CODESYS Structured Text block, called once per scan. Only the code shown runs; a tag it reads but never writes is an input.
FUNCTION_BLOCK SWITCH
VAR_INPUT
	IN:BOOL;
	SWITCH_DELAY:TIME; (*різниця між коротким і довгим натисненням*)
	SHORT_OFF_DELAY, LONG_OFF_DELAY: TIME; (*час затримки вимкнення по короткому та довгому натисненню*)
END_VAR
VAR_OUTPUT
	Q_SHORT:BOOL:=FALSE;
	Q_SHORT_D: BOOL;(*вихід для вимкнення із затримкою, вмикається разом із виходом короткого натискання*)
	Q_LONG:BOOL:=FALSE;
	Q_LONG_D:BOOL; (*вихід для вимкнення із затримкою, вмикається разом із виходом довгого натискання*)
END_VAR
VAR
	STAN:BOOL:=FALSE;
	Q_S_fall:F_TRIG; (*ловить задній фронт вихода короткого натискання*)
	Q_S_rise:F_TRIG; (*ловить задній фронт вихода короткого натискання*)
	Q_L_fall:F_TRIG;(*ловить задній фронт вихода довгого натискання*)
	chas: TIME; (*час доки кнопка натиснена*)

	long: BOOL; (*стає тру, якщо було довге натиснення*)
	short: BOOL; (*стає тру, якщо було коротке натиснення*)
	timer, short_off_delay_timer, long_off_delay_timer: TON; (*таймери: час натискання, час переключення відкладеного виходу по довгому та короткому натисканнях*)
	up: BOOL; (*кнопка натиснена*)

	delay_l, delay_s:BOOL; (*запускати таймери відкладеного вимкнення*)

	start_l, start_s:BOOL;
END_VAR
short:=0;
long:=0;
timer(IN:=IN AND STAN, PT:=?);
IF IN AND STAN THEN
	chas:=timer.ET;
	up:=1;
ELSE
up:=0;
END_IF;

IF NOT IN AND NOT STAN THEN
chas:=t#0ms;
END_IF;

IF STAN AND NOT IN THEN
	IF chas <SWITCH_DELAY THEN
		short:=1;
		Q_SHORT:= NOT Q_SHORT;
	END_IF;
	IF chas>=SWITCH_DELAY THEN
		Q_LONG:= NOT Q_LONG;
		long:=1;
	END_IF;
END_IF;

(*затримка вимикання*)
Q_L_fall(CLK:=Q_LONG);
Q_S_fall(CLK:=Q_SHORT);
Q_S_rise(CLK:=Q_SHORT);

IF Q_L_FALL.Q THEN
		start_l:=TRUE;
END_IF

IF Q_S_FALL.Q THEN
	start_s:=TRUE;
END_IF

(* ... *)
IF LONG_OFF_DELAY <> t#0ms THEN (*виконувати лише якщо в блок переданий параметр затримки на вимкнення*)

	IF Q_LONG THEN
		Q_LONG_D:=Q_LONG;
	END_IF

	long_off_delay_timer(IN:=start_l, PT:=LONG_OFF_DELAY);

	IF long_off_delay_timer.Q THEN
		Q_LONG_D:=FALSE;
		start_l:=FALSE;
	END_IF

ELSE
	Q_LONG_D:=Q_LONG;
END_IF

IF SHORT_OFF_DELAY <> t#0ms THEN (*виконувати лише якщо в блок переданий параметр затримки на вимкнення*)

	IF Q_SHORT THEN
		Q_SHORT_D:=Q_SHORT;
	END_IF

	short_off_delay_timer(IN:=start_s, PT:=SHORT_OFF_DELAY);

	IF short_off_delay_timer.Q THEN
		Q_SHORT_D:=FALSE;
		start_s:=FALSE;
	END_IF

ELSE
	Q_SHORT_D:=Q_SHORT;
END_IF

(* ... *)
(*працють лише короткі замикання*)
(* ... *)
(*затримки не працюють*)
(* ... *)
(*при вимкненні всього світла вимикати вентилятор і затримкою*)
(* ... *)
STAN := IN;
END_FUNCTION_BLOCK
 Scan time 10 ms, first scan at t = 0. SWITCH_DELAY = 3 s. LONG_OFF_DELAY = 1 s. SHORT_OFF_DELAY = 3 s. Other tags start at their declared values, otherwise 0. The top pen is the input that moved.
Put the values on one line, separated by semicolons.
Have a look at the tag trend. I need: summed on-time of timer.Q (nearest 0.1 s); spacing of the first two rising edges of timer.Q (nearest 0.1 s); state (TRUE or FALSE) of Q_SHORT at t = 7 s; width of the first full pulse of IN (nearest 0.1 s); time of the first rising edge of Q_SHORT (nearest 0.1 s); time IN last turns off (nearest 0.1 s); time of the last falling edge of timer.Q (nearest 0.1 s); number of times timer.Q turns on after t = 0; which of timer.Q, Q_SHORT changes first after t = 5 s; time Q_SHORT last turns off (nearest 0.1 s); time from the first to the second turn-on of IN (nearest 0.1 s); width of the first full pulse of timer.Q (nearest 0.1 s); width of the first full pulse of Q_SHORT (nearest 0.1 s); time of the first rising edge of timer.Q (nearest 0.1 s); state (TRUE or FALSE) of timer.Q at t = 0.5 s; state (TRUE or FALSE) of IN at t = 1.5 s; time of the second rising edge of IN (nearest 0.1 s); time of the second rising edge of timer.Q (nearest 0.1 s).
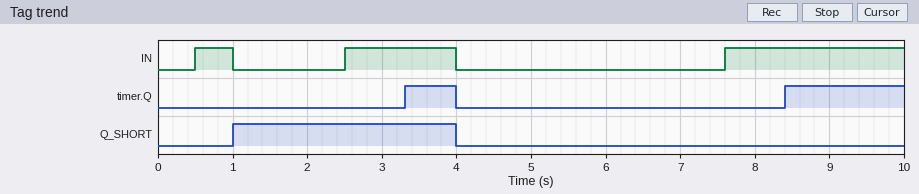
2.3 s; 5.1 s; FALSE; 0.5 s; 1.0 s; 4.0 s; 4.0 s; 2; timer.Q; 4.0 s; 2.0 s; 0.7 s; 3.0 s; 3.3 s; FALSE; FALSE; 2.5 s; 8.4 s
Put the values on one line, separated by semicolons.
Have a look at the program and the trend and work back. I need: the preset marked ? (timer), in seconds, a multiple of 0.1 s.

0.8 s
